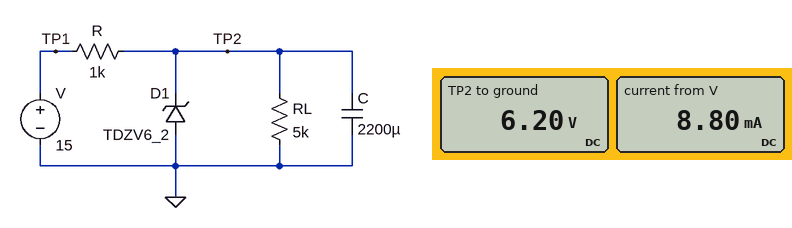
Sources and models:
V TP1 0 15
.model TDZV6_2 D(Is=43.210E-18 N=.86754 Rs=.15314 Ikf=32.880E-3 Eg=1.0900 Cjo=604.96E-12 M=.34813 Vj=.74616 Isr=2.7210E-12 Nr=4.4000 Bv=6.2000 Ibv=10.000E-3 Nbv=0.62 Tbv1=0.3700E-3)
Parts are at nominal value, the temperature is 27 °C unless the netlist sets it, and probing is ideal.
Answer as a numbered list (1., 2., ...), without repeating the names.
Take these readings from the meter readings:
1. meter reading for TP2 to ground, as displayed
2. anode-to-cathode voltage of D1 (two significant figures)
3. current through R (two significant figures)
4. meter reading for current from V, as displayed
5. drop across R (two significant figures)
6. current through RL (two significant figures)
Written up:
1. 6.20 V
2. -6.2 V
3. 8.8 mA
4. 8.80 mA
5. 8.8 V
6. 1.2 mA
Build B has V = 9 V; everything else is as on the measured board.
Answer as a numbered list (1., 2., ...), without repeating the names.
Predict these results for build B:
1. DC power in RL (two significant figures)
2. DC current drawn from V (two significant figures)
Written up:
1. 7.6 mW
2. 2.8 mA
